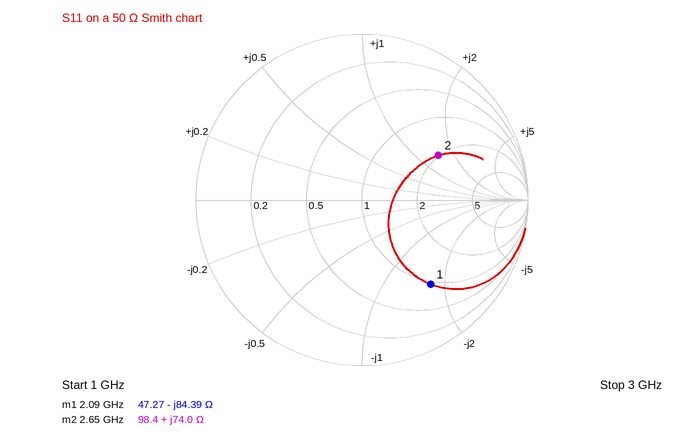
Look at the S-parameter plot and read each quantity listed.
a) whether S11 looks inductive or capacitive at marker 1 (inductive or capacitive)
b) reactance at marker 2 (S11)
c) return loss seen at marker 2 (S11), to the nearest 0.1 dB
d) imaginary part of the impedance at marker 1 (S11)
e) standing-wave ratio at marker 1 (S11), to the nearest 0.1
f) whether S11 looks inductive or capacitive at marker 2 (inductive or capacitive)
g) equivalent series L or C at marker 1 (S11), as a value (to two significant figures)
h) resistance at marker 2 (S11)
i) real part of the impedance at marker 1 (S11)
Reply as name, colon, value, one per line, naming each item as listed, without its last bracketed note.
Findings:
whether S11 looks inductive or capacitive at marker 1: capacitive
reactance at marker 2: +74.0 Ω
return loss seen at marker 2 (S11), to the nearest 0.1 dB: 5.5 dB
imaginary part of the impedance at marker 1: -84.39 Ω
standing-wave ratio at marker 1 (S11), to the nearest 0.1: 4.8
whether S11 looks inductive or capacitive at marker 2: inductive
equivalent series L or C at marker 1 (S11), as a value: 900 fF
resistance at marker 2: 98.4 Ω
real part of the impedance at marker 1: 47.27 Ω
